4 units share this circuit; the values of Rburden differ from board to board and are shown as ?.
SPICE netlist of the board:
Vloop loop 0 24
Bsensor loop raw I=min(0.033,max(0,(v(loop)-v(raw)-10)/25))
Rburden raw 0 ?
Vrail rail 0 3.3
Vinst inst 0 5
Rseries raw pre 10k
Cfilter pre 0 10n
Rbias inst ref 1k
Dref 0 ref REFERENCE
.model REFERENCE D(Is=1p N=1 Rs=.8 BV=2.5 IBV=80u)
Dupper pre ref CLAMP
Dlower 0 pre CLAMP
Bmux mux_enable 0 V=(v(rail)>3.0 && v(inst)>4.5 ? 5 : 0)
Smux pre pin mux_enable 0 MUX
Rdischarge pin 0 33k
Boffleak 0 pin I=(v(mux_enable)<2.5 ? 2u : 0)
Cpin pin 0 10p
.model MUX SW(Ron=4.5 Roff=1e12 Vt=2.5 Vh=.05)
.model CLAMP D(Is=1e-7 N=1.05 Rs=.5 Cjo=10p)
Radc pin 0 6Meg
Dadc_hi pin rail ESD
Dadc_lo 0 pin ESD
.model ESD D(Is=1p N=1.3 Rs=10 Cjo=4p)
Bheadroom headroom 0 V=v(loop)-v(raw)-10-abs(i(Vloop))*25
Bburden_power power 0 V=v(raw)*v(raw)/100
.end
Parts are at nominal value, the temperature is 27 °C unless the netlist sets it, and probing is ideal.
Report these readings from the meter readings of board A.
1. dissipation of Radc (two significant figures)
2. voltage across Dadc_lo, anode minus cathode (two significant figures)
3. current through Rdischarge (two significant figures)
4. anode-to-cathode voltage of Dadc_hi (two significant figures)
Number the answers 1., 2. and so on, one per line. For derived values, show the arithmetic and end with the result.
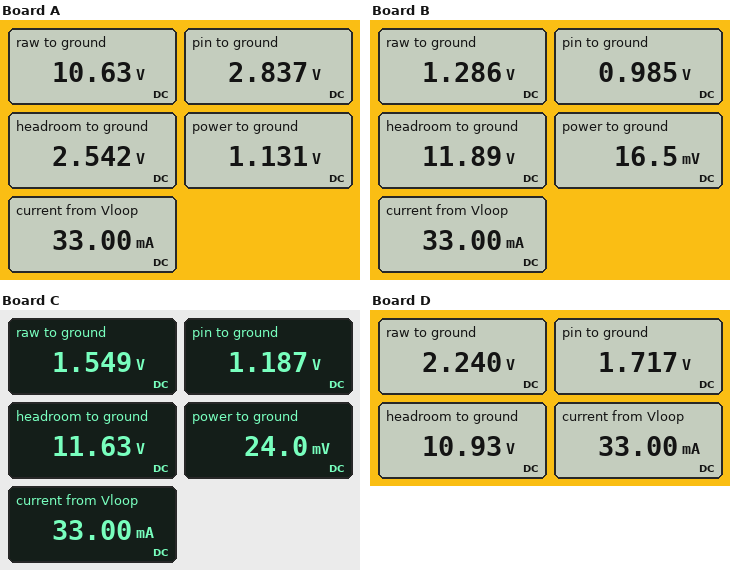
1. (2.837 V)^2 / 6 MΩ = 1.3 µW
2. 0 V - 2.837 V = -2.8 V
3. (2.837 V) / 33 kΩ = 86 µA
4. 2.837 V - 3.3 V = -460 mV
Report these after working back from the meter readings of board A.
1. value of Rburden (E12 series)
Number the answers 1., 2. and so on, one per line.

1. 330 Ω
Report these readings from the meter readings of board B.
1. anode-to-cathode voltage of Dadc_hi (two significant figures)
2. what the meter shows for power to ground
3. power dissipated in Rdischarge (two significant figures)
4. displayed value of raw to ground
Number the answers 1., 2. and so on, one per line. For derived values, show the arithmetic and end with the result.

1. 985 mV - 3.3 V = -2.3 V
2. 16.5 mV
3. (985 mV)^2 / 33 kΩ = 29 µW
4. 1.286 V
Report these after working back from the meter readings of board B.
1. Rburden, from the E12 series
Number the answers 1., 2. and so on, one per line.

1. 39 Ω
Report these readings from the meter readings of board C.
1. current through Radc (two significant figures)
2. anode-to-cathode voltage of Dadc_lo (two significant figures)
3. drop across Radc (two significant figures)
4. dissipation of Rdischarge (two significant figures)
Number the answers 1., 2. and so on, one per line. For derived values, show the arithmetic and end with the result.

1. (1.187 V) / 6 MΩ = 200 nA
2. 0 V - 1.187 V = -1.2 V
3. 1.187 V = 1.2 V
4. (1.187 V)^2 / 33 kΩ = 43 µW
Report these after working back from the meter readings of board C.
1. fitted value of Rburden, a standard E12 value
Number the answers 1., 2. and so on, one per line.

1. 47 Ω
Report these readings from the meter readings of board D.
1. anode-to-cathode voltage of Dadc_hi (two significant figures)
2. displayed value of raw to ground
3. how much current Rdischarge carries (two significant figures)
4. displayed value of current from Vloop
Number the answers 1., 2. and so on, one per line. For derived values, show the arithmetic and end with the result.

1. 1.717 V - 3.3 V = -1.6 V
2. 2.240 V
3. (1.717 V) / 33 kΩ = 52 µA
4. 33.00 mA
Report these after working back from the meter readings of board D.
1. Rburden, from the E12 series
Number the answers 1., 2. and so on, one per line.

1. 68 Ω
